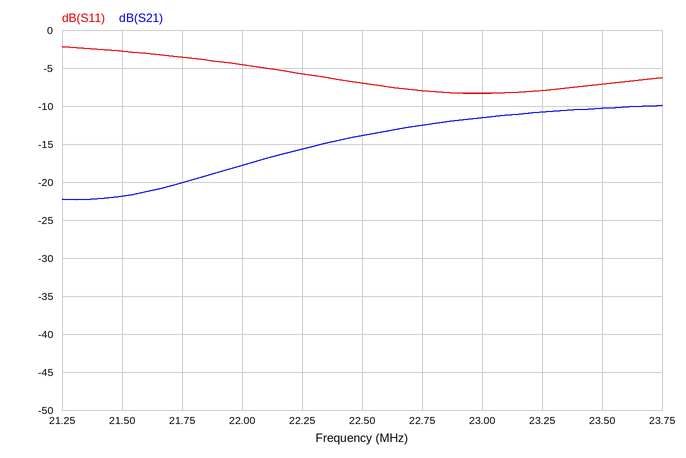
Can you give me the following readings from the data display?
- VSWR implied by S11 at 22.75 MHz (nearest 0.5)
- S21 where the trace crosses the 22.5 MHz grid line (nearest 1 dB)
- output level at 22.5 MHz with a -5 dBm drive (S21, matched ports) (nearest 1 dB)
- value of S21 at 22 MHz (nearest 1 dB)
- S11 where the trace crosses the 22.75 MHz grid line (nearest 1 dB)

2.5
-14 dB
-19 dBm
-18 dB
-8 dB
